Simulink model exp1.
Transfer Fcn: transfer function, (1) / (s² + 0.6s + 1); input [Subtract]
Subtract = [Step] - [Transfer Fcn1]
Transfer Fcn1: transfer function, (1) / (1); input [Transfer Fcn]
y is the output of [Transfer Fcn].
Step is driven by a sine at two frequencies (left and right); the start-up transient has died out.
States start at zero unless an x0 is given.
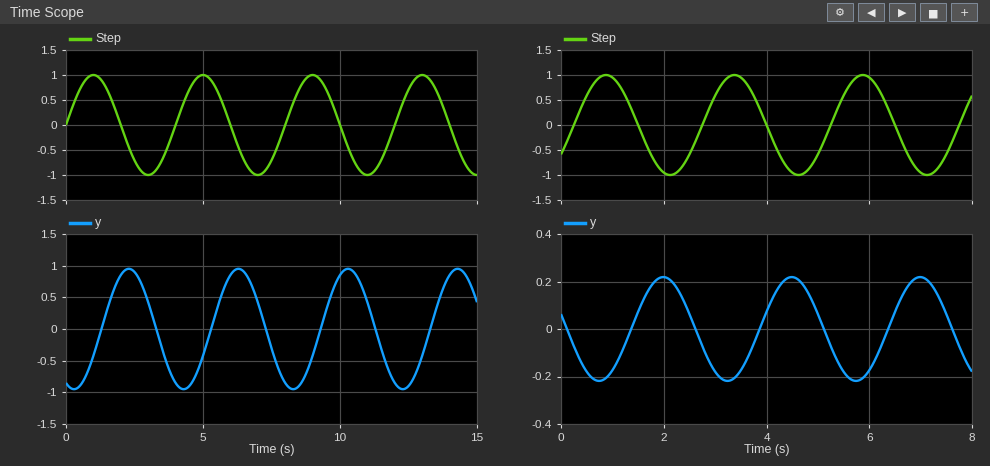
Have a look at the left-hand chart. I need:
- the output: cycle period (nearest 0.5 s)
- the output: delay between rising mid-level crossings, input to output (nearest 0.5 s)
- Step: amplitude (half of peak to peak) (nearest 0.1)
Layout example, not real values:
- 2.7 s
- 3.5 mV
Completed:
- 4.0 s
- 1.5 s
- 1.0
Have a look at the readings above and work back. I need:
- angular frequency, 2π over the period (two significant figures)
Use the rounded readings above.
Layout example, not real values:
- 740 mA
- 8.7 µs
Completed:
- 1.6 rad/s
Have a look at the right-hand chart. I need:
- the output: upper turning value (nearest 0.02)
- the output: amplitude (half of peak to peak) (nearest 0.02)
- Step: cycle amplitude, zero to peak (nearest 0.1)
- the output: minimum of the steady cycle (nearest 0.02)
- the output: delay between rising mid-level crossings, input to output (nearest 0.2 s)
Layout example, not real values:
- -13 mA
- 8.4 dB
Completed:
- 0.22
- 0.22
- 1.0
- -0.22
- 1.2 s
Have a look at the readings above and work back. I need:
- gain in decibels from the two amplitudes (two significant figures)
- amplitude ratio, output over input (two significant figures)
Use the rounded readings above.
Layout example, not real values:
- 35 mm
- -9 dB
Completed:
- -13 dB
- 0.22
